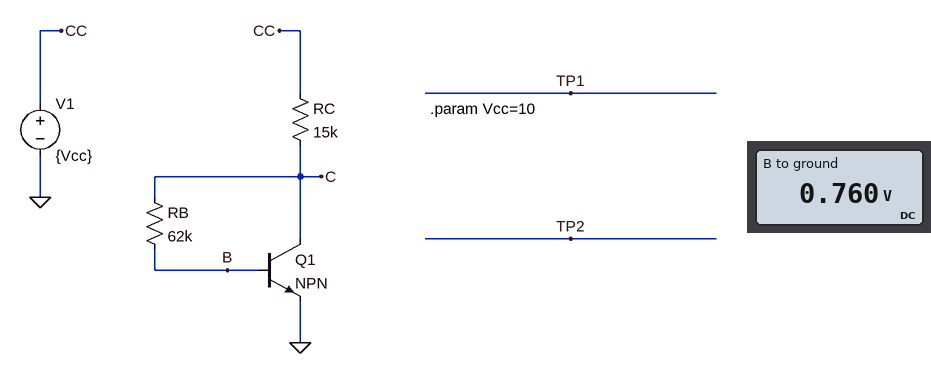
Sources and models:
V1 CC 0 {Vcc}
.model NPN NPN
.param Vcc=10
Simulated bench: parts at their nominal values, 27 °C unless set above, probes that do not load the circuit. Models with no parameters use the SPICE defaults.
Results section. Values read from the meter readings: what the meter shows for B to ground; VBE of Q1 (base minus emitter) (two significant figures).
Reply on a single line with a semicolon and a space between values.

0.760 V; 760 mV
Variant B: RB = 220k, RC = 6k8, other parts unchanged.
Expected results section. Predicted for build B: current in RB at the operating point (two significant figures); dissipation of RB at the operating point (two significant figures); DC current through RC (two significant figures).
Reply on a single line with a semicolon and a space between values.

10 µA; 23 µW; 1.0 mA
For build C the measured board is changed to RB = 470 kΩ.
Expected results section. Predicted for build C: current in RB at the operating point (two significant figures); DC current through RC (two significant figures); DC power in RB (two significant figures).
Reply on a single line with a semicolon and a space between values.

4.7 µA; 470 µA; 10 µW
